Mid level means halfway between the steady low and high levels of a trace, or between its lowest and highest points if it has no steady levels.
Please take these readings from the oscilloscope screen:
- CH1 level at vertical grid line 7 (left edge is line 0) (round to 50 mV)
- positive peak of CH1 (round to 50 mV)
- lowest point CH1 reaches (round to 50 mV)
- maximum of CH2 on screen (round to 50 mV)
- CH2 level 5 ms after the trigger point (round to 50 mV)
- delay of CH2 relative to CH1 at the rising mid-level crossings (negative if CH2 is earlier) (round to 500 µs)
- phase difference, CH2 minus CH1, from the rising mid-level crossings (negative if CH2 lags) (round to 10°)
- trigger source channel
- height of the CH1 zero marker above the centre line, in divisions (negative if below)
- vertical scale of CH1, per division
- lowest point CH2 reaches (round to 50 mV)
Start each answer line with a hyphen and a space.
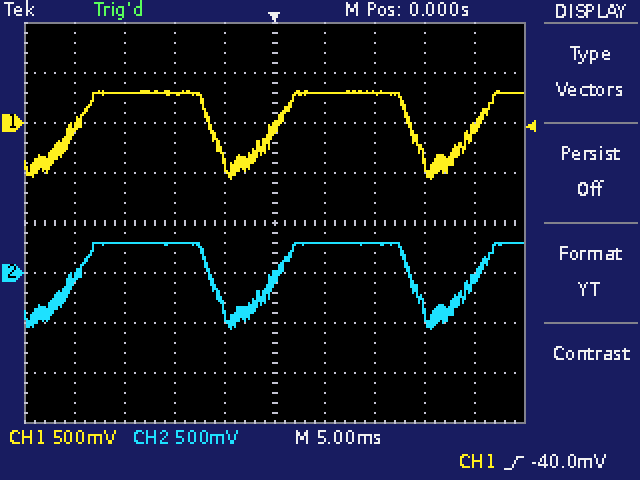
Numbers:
- 300 mV
- 300 mV
- -550 mV
- 300 mV
- 300 mV
- 0.0 ms
- 0°
- CH1
- +2.0 div
- 500 mV
- -550 mV
